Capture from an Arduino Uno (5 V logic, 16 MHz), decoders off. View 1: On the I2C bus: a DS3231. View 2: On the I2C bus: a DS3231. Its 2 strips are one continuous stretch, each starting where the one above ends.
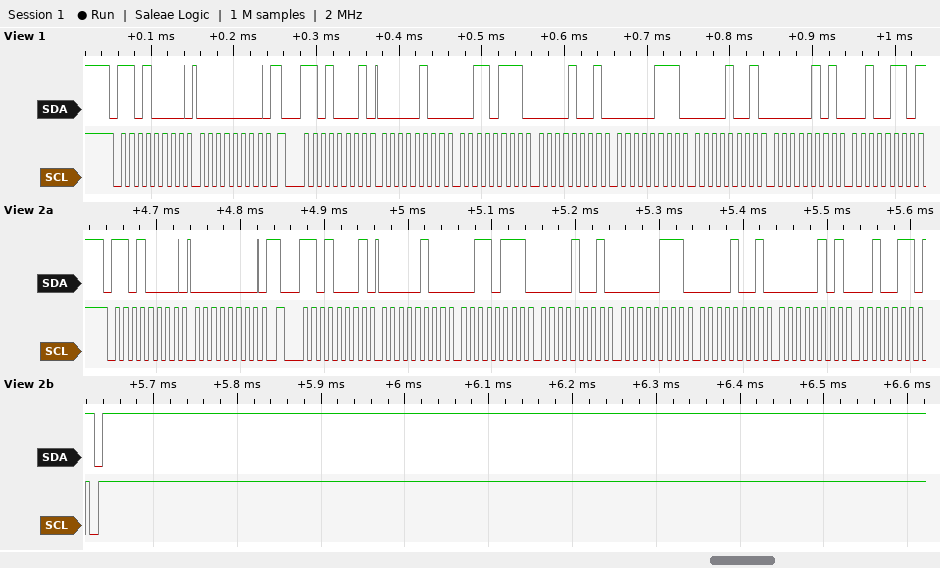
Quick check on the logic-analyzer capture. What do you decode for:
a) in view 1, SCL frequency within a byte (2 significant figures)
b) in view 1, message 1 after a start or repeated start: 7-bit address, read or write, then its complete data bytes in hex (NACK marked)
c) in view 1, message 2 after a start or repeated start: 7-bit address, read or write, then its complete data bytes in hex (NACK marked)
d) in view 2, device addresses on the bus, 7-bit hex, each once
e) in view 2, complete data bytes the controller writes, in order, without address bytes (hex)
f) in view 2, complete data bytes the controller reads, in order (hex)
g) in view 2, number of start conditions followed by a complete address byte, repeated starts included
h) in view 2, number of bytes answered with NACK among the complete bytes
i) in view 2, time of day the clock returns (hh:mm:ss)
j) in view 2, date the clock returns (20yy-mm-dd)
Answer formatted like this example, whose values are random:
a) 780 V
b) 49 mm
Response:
a) 100 kHz
b) 0x68 write: 00
c) 0x68 read: 04 37 09 07 09 05 26 NACK
d) 0x68
e) 00
f) 04 37 09 07 09 05 26
g) 2
h) 1
i) 09:37:04
j) 2026-05-09
